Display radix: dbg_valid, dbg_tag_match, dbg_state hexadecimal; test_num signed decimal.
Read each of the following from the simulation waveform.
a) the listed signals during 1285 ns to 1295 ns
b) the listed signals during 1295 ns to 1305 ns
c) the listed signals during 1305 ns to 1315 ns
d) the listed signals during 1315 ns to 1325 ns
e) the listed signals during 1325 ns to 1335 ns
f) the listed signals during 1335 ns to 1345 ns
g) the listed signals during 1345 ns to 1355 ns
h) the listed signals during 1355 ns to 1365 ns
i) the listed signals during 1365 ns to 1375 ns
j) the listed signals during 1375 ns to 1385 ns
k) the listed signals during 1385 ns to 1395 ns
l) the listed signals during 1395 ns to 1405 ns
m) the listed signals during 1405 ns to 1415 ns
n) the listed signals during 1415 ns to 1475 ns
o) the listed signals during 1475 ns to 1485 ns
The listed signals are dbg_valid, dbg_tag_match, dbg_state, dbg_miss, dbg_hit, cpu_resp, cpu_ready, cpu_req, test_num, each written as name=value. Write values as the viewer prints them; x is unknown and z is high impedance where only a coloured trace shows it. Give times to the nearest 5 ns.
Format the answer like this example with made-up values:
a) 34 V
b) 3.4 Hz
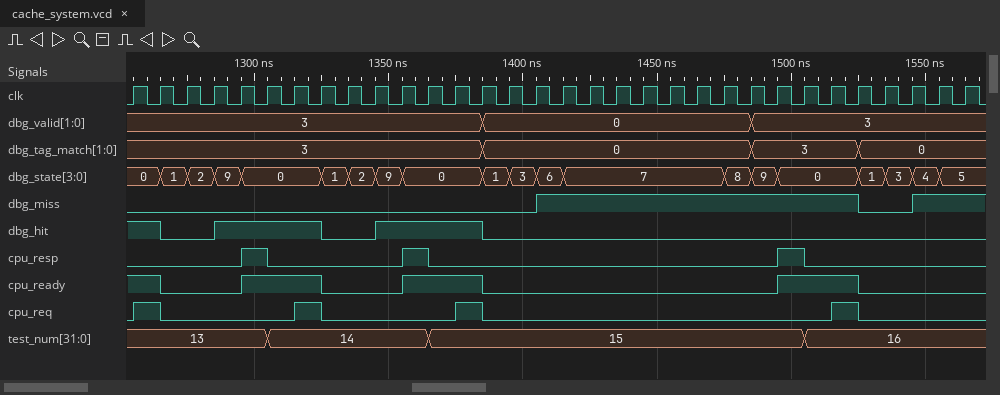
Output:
a) dbg_valid=3, dbg_tag_match=3, dbg_state=9, dbg_miss=0, dbg_hit=1, cpu_resp=0, cpu_ready=0, cpu_req=0, test_num=13
b) dbg_valid=3, dbg_tag_match=3, dbg_state=0, dbg_miss=0, dbg_hit=1, cpu_resp=1, cpu_ready=1, cpu_req=0, test_num=13
c) dbg_valid=3, dbg_tag_match=3, dbg_state=0, dbg_miss=0, dbg_hit=1, cpu_resp=0, cpu_ready=1, cpu_req=0, test_num=14
d) dbg_valid=3, dbg_tag_match=3, dbg_state=0, dbg_miss=0, dbg_hit=1, cpu_resp=0, cpu_ready=1, cpu_req=1, test_num=14
e) dbg_valid=3, dbg_tag_match=3, dbg_state=1, dbg_miss=0, dbg_hit=0, cpu_resp=0, cpu_ready=0, cpu_req=0, test_num=14
f) dbg_valid=3, dbg_tag_match=3, dbg_state=2, dbg_miss=0, dbg_hit=0, cpu_resp=0, cpu_ready=0, cpu_req=0, test_num=14
g) dbg_valid=3, dbg_tag_match=3, dbg_state=9, dbg_miss=0, dbg_hit=1, cpu_resp=0, cpu_ready=0, cpu_req=0, test_num=14
h) dbg_valid=3, dbg_tag_match=3, dbg_state=0, dbg_miss=0, dbg_hit=1, cpu_resp=1, cpu_ready=1, cpu_req=0, test_num=14
i) dbg_valid=3, dbg_tag_match=3, dbg_state=0, dbg_miss=0, dbg_hit=1, cpu_resp=0, cpu_ready=1, cpu_req=0, test_num=15
j) dbg_valid=3, dbg_tag_match=3, dbg_state=0, dbg_miss=0, dbg_hit=1, cpu_resp=0, cpu_ready=1, cpu_req=1, test_num=15
k) dbg_valid=0, dbg_tag_match=0, dbg_state=1, dbg_miss=0, dbg_hit=0, cpu_resp=0, cpu_ready=0, cpu_req=0, test_num=15
l) dbg_valid=0, dbg_tag_match=0, dbg_state=3, dbg_miss=0, dbg_hit=0, cpu_resp=0, cpu_ready=0, cpu_req=0, test_num=15
m) dbg_valid=0, dbg_tag_match=0, dbg_state=6, dbg_miss=1, dbg_hit=0, cpu_resp=0, cpu_ready=0, cpu_req=0, test_num=15
n) dbg_valid=0, dbg_tag_match=0, dbg_state=7, dbg_miss=1, dbg_hit=0, cpu_resp=0, cpu_ready=0, cpu_req=0, test_num=15
o) dbg_valid=0, dbg_tag_match=0, dbg_state=8, dbg_miss=1, dbg_hit=0, cpu_resp=0, cpu_ready=0, cpu_req=0, test_num=15
